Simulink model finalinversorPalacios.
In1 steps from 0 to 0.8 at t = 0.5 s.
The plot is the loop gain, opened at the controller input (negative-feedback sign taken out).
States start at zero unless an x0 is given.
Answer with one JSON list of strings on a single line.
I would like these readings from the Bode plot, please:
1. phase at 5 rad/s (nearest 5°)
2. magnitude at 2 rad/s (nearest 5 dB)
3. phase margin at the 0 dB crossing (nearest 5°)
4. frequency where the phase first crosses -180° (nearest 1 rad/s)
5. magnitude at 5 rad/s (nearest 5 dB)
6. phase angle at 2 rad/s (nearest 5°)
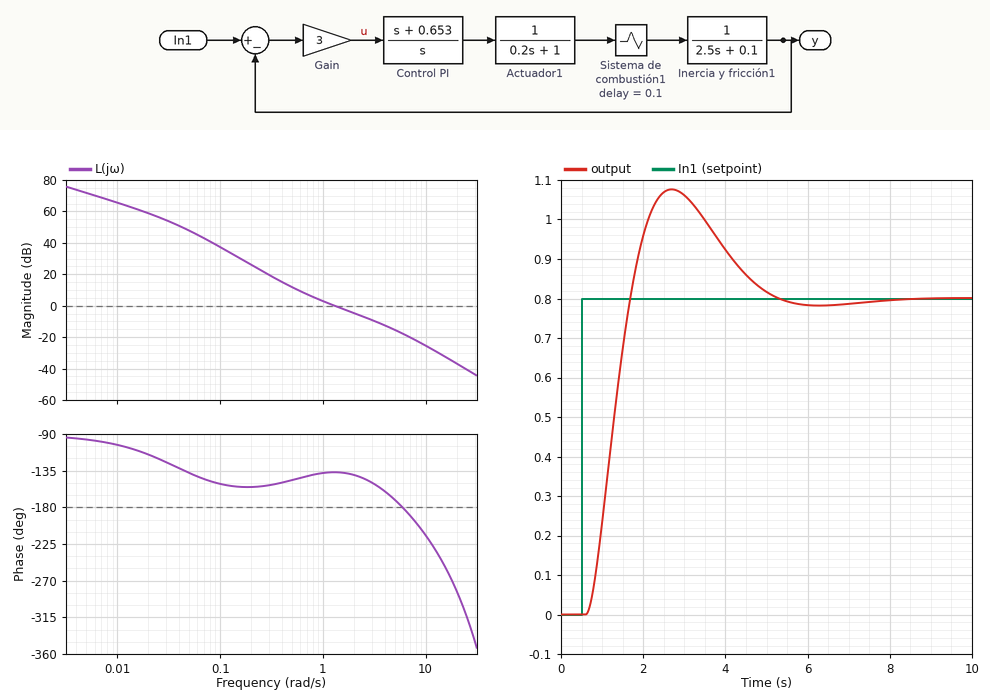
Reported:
["-170°", "-5 dB", "45°", "6 rad/s", "-15 dB", "-140°"]
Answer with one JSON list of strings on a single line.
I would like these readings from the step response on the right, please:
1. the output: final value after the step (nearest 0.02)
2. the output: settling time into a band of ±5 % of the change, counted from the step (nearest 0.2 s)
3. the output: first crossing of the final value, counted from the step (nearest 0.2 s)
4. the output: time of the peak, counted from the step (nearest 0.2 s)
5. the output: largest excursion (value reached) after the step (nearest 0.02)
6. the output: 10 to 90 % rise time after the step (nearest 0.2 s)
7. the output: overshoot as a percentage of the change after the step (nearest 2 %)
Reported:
["0.80", "4.2 s", "1.2 s", "2.2 s", "1.08", "0.8 s", "34 %"]
